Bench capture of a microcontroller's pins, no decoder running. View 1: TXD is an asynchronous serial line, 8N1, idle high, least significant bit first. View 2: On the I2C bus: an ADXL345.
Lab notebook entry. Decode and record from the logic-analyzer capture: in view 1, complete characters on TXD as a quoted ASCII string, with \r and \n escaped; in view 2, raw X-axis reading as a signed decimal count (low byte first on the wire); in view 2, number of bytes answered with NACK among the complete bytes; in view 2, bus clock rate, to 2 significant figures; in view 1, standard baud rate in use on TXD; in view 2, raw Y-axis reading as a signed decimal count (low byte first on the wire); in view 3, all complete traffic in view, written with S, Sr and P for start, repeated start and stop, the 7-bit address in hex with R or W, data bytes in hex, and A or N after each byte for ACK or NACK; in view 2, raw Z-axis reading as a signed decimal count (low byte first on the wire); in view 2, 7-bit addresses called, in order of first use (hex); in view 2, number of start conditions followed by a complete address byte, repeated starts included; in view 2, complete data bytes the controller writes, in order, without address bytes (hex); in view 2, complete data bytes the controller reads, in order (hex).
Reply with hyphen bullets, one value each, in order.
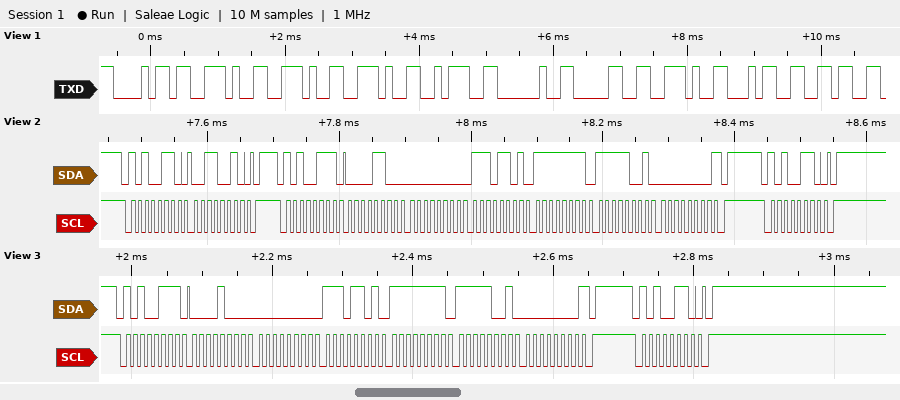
- "h...: 0.46"
- 12
- 1
- 100 kHz
- 9600 baud
- -19
- S 53R A 08 A 00 A ED A FF A F9 A 00 N P S 53W A P
- 249
- 0x53
- 3
- 32
- 0C 00 ED FF F9 00
